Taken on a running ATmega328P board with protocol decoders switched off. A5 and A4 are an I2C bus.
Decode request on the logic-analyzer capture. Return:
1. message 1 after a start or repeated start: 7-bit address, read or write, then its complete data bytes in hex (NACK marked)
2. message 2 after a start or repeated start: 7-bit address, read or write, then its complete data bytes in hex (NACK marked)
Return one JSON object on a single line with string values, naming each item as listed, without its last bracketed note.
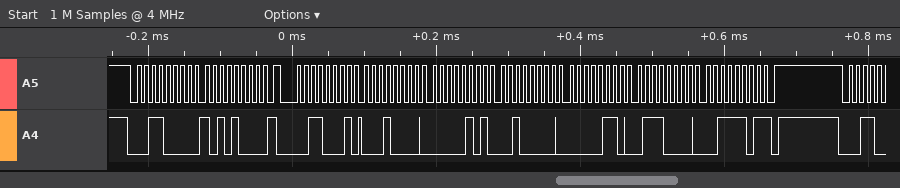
{"message 1 after a start or repeated start: 7-bit address, read or write, then its complete data bytes in hex": "0x18 write: A8", "message 2 after a start or repeated start: 7-bit address, read or write, then its complete data bytes in hex": "0x18 read: 10 05 20 06 70 3D NACK"}
